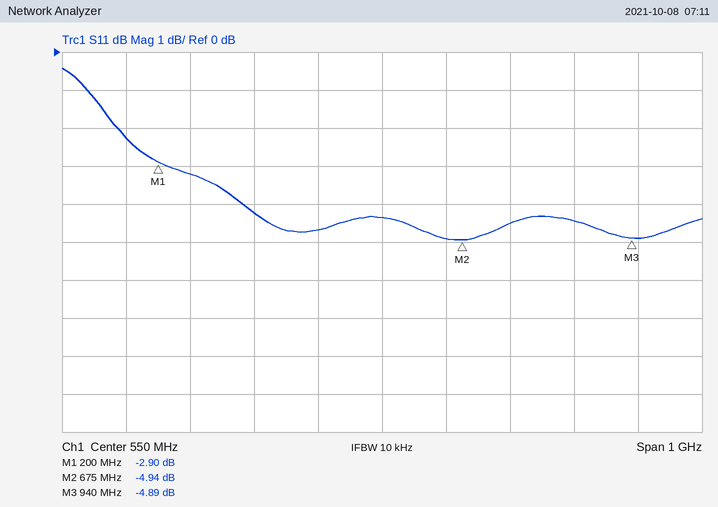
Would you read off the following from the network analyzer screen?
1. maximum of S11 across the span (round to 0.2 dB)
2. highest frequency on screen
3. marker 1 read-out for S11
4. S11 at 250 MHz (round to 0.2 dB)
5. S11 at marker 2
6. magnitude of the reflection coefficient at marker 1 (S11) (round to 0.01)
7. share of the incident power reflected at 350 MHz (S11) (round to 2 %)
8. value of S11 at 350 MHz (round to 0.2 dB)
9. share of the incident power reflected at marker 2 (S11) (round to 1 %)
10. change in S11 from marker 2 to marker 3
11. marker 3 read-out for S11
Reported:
-0.4 dB
1.05 GHz
-2.90 dB
-3.2 dB
-4.94 dB
0.72
38 %
-4.2 dB
32 %
0.05 dB
-4.89 dB
